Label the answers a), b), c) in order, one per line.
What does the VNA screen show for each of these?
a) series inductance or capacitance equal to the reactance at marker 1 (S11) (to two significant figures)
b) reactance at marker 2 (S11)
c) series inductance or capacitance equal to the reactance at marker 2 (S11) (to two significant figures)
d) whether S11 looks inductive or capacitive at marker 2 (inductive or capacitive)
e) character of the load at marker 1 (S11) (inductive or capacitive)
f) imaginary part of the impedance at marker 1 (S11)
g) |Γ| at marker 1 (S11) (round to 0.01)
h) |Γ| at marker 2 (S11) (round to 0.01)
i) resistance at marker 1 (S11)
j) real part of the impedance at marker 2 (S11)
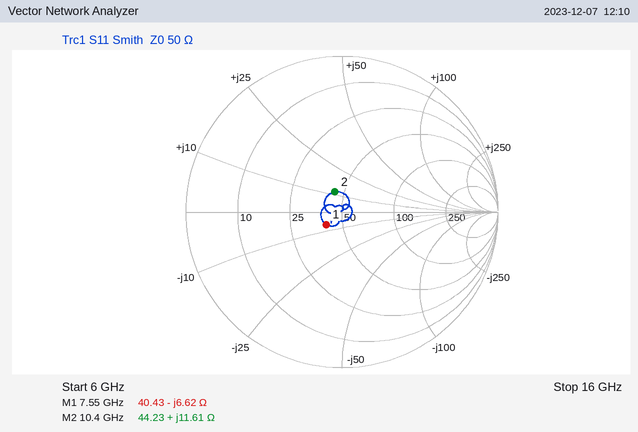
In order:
a) 3.2 pF
b) +11.61 Ω
c) 180 pH
d) inductive
e) capacitive
f) -6.62 Ω
g) 0.13
h) 0.14
i) 40.43 Ω
j) 44.23 Ω
